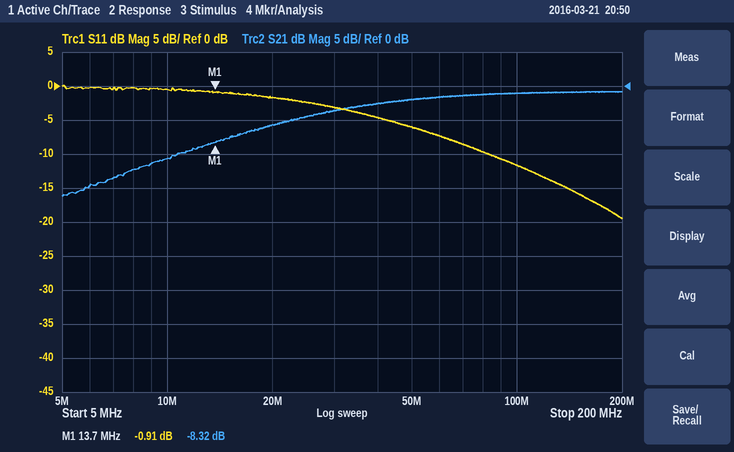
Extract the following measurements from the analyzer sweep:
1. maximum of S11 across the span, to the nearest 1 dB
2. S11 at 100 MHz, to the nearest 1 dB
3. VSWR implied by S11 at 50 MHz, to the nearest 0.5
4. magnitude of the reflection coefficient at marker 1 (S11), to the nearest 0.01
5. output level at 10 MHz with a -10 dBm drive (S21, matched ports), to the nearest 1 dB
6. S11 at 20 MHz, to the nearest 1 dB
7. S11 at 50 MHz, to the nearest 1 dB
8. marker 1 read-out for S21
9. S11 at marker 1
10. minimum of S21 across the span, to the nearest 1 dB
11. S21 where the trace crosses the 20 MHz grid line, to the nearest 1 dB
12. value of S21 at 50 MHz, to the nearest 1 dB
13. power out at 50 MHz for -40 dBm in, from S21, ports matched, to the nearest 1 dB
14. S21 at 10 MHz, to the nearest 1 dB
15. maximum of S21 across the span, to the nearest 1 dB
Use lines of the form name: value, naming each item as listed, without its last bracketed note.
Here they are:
maximum of S11 across the span, to the nearest 1 dB: 0 dB
S11 at 100 MHz, to the nearest 1 dB: -12 dB
VSWR implied by S11 at 50 MHz, to the nearest 0.5: 3.0
magnitude of the reflection coefficient at marker 1 (S11), to the nearest 0.01: 0.90
output level at 10 MHz with a -10 dBm drive (S21, matched ports), to the nearest 1 dB: -21 dBm
S11 at 20 MHz, to the nearest 1 dB: -2 dB
S11 at 50 MHz, to the nearest 1 dB: -6 dB
marker 1 read-out for S21: -8.32 dB
S11 at marker 1: -0.91 dB
minimum of S21 across the span, to the nearest 1 dB: -16 dB
S21 where the trace crosses the 20 MHz grid line, to the nearest 1 dB: -6 dB
value of S21 at 50 MHz, to the nearest 1 dB: -2 dB
power out at 50 MHz for -40 dBm in, from S21, ports matched, to the nearest 1 dB: -42 dBm
S21 at 10 MHz, to the nearest 1 dB: -11 dB
maximum of S21 across the span, to the nearest 1 dB: -1 dB
